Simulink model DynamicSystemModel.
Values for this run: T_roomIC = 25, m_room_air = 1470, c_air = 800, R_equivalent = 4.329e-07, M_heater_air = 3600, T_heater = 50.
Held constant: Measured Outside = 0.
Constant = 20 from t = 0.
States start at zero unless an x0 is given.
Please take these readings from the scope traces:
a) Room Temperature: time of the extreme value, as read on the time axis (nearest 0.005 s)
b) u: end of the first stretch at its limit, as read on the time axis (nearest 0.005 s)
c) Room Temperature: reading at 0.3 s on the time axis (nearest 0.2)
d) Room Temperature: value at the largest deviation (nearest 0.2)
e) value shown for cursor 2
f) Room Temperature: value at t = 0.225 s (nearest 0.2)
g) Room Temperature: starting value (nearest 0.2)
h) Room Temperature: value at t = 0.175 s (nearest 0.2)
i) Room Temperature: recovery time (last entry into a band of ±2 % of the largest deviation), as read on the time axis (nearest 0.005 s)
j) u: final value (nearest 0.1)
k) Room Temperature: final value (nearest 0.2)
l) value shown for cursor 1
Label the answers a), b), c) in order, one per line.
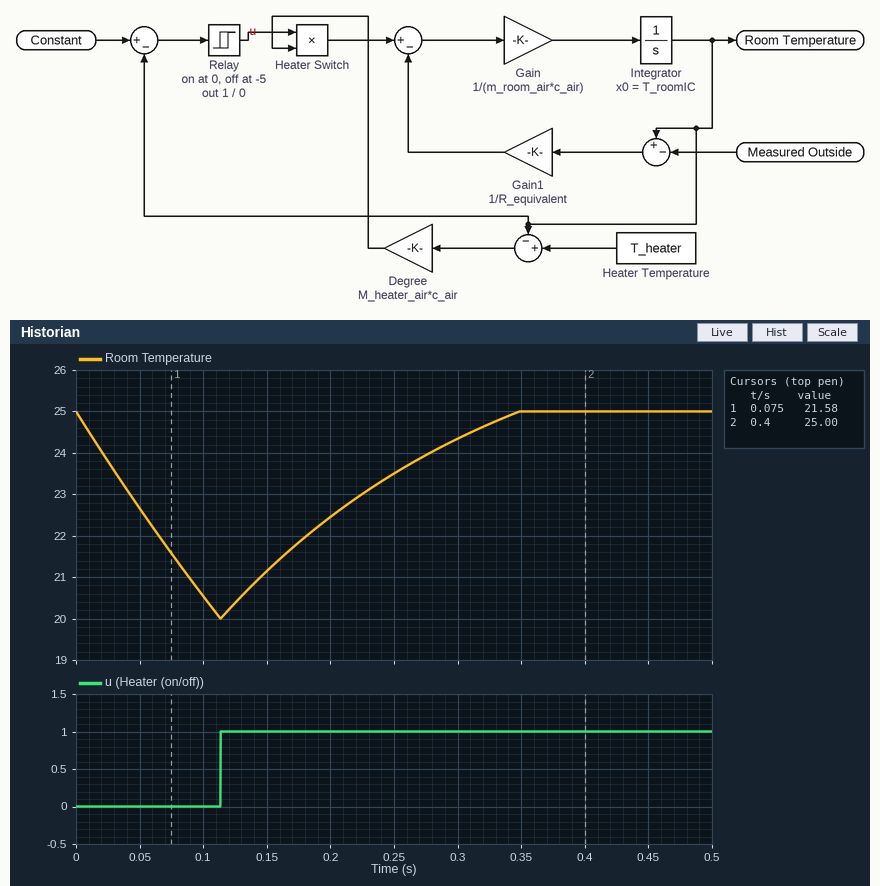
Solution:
a) 0.115 s
b) 0.115 s
c) 24.4
d) 20.0
e) 25.00
f) 23.0
g) 25.0
h) 21.8
i) 0.340 s
j) 1.0
k) 25.0
l) 21.58
